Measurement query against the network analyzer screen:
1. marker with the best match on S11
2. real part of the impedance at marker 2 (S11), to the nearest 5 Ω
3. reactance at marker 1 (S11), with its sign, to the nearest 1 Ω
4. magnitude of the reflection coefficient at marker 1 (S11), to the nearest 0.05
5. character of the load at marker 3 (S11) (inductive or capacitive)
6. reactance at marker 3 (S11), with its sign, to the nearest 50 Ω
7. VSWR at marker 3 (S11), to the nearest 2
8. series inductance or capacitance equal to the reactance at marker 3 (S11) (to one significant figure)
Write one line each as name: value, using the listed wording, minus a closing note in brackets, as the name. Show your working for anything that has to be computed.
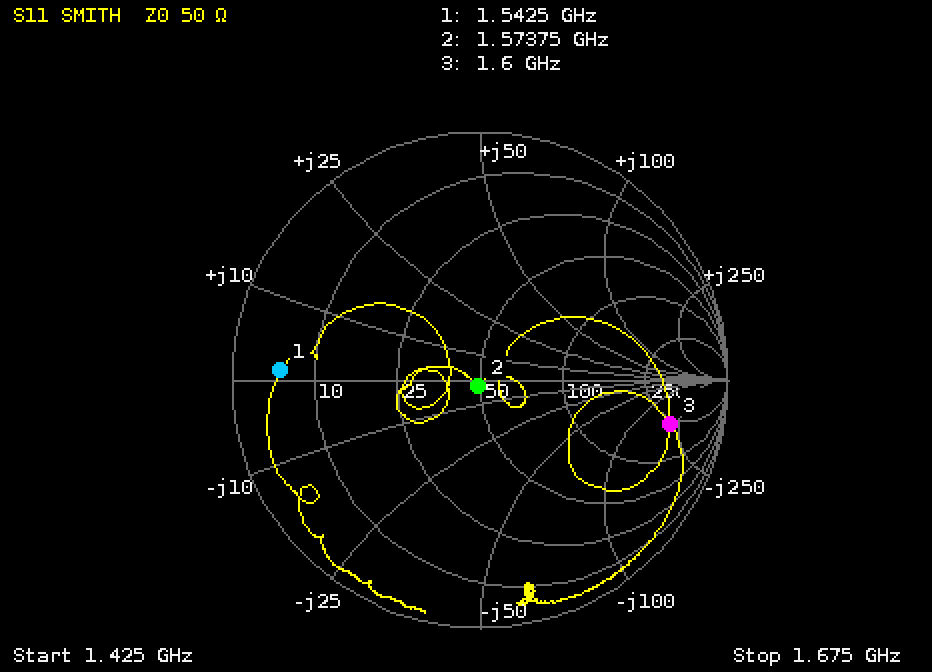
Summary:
marker with the best match on S11: marker 2
real part of the impedance at marker 2 (S11), to the nearest 5 Ω: 50 Ω
reactance at marker 1 (S11), with its sign, to the nearest 1 Ω: +1 Ω
magnitude of the reflection coefficient at marker 1 (S11), to the nearest 0.05: 0.80
character of the load at marker 3 (S11): capacitive
reactance at marker 3 (S11), with its sign, to the nearest 50 Ω: -200 Ω
VSWR at marker 3 (S11), to the nearest 2: 8
series inductance or capacitance equal to the reactance at marker 3 (S11): C = 1/(2π × 1.6 GHz × 200 Ω) ≈ 497 fF, so 500 fF to one significant figure
